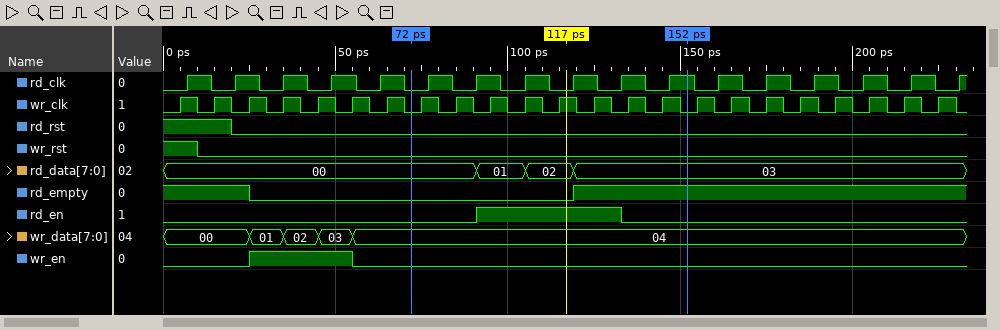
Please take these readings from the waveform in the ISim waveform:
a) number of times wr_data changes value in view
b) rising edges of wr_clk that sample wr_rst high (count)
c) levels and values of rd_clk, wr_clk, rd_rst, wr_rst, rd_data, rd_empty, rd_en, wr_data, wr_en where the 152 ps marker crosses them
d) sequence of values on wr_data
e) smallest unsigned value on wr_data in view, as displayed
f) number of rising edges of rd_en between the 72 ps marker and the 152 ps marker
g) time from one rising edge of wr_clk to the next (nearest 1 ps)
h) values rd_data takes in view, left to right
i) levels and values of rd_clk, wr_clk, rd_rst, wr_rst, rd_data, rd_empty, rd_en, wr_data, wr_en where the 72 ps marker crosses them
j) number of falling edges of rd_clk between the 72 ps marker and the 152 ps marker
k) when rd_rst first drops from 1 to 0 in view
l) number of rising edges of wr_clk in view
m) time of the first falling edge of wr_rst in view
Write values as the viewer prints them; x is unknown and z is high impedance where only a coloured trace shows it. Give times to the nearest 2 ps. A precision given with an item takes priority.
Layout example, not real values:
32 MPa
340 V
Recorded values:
4
1
rd_clk=1, wr_clk=0, rd_rst=0, wr_rst=0, rd_data=03, rd_empty=1, rd_en=0, wr_data=04, wr_en=0
00, 01, 02, 03, 04
00
1
10 ps
00, 01, 02, 03
rd_clk=0, wr_clk=0, rd_rst=0, wr_rst=0, rd_data=00, rd_empty=0, rd_en=0, wr_data=04, wr_en=0
5
20 ps
23
10 ps
